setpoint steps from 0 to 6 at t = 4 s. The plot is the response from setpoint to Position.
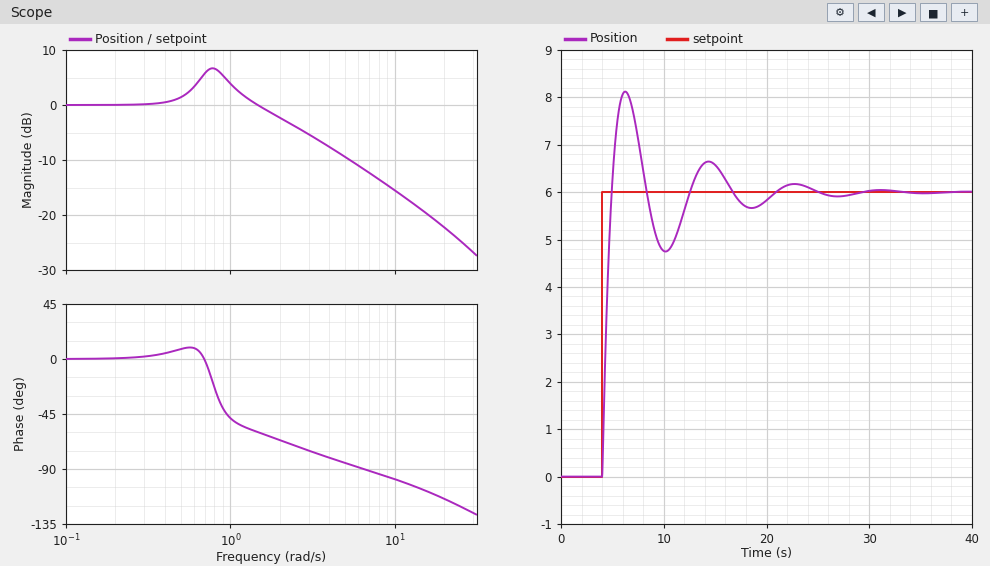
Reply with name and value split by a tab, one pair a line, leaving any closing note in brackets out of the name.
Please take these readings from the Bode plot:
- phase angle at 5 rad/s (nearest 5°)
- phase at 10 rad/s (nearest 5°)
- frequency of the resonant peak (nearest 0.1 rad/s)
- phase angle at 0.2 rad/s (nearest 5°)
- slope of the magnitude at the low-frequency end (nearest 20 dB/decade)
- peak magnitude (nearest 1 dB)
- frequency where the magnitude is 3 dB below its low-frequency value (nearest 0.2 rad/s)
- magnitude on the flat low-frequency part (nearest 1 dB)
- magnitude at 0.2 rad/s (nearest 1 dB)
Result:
phase angle at 5 rad/s	-85°
phase at 10 rad/s	-100°
frequency of the resonant peak	0.8 rad/s
phase angle at 0.2 rad/s	0°
slope of the magnitude at the low-frequency end	0 dB/decade
peak magnitude	7 dB
frequency where the magnitude is 3 dB below its low-frequency value	2.2 rad/s
magnitude on the flat low-frequency part	0 dB
magnitude at 0.2 rad/s	0 dB
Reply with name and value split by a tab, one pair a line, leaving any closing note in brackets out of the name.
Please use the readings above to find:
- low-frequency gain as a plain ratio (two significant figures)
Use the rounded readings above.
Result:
low-frequency gain as a plain ratio	1.0
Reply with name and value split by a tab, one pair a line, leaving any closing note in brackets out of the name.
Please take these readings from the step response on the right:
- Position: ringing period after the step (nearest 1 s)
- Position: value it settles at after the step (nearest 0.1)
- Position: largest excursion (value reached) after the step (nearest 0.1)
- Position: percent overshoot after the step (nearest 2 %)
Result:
Position: ringing period after the step	8 s
Position: value it settles at after the step	6.0
Position: largest excursion (value reached) after the step	8.1
Position: percent overshoot after the step	36 %
